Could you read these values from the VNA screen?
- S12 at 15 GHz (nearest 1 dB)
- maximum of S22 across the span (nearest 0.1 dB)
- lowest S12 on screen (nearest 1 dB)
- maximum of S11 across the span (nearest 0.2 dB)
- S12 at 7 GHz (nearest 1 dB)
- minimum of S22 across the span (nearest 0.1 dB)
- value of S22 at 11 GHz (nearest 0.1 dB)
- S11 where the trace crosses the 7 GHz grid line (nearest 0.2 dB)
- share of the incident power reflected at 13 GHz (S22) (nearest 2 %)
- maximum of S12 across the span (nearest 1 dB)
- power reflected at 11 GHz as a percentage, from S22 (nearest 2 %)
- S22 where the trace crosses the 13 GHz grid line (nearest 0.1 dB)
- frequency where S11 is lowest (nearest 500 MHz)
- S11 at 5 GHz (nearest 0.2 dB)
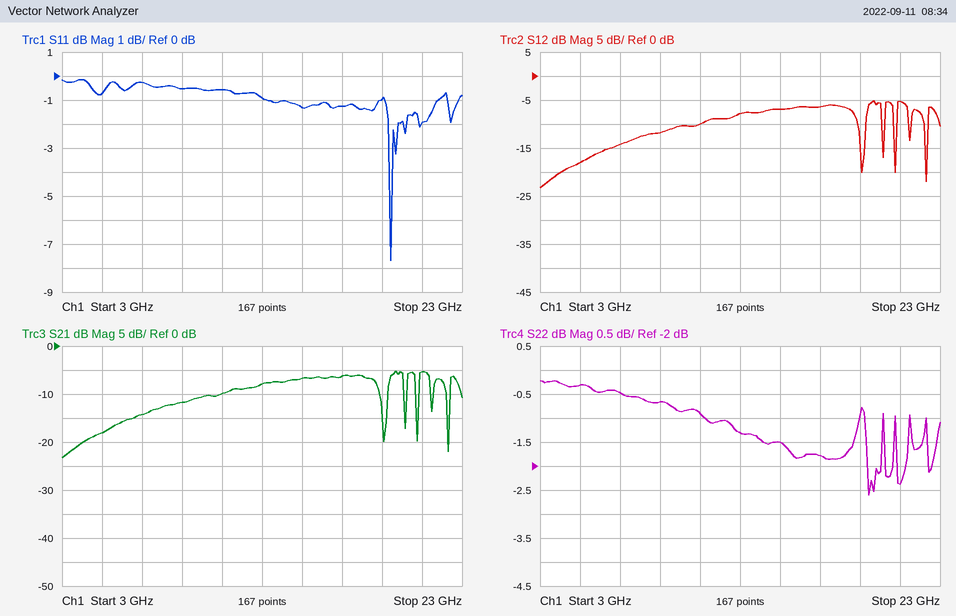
-7 dB
-0.2 dB
-23 dB
-0.2 dB
-14 dB
-2.6 dB
-0.9 dB
-0.2 dB
74 %
-5 dB
82 %
-1.3 dB
19.5 GHz
-0.8 dB
